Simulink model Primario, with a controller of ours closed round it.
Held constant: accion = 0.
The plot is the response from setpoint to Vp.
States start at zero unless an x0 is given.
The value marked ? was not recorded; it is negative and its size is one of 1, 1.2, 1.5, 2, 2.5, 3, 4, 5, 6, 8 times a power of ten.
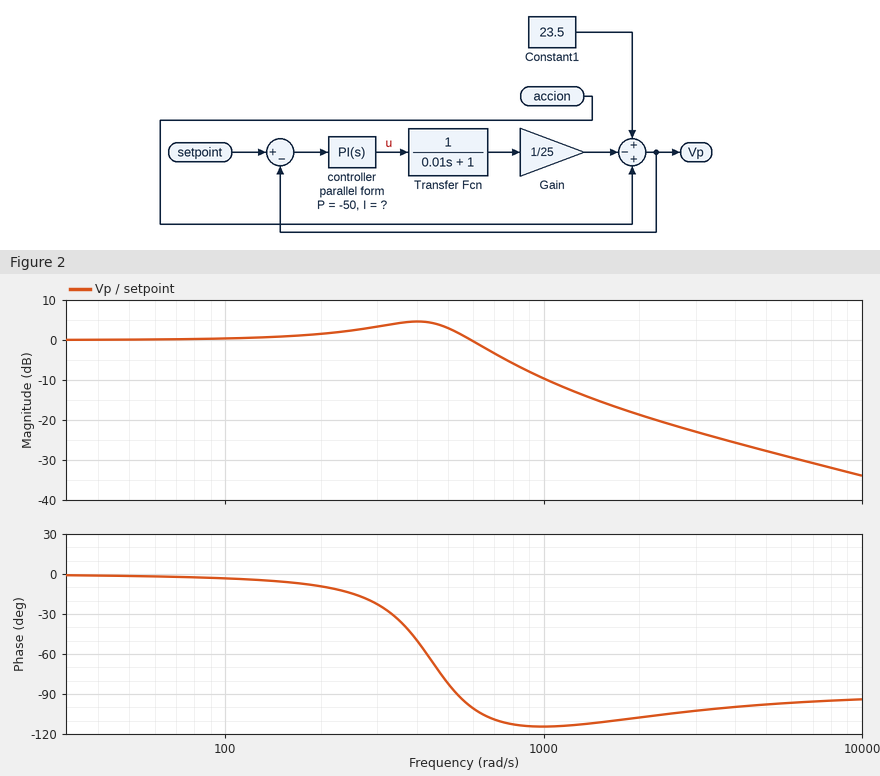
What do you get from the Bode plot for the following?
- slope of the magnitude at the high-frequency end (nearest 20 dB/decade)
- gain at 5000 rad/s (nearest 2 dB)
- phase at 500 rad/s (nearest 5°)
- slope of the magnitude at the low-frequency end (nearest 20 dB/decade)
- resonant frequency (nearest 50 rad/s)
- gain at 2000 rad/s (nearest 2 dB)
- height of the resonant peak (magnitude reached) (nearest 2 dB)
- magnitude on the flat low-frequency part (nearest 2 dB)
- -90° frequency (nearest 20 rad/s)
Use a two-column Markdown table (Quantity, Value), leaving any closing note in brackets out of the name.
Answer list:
| Quantity | Value |
|---|---|
| slope of the magnitude at the high-frequency end | -20 dB/decade |
| gain at 5000 rad/s | -28 dB |
| phase at 500 rad/s | -80° |
| slope of the magnitude at the low-frequency end | 0 dB/decade |
| resonant frequency | 400 rad/s |
| gain at 2000 rad/s | -18 dB |
| height of the resonant peak (magnitude reached) | 4 dB |
| magnitude on the flat low-frequency part | 0 dB |
| -90° frequency | 540 rad/s |
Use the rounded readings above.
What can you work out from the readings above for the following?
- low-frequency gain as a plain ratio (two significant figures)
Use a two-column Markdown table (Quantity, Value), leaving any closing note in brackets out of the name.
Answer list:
| Quantity | Value |
|---|---|
| low-frequency gain as a plain ratio | 1.0 |
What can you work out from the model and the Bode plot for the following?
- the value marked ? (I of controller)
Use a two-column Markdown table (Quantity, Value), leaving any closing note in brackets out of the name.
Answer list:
| Quantity | Value |
|---|---|
| the value marked ? | -50000 |
